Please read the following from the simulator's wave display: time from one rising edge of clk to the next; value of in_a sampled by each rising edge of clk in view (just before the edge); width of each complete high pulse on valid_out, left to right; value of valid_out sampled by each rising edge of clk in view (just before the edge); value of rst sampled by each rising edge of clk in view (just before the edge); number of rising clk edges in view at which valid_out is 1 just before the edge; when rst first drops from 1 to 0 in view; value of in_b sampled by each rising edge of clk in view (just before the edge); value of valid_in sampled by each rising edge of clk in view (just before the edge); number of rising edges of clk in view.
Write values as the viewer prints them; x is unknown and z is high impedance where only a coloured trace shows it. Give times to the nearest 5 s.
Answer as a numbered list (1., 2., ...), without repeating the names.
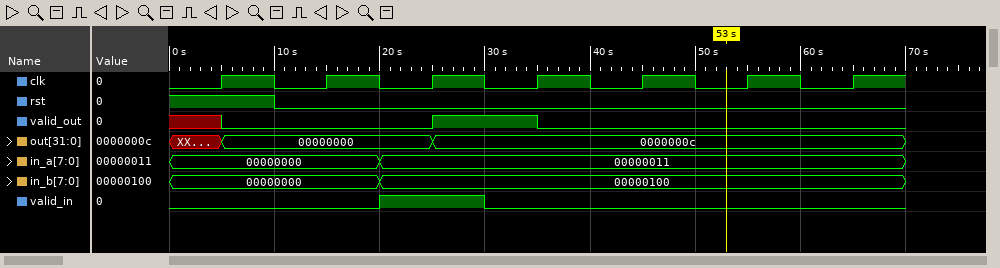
1. 10 s
2. 00000000, 00000000, 00000011, 00000011, 00000011, 00000011, 00000011
3. 10 s
4. x 0 0 1 0 0 0
5. 1 0 0 0 0 0 0
6. 1
7. 10 s
8. 00000000, 00000000, 00000100, 00000100, 00000100, 00000100, 00000100
9. 0 0 1 0 0 0 0
10. 7
